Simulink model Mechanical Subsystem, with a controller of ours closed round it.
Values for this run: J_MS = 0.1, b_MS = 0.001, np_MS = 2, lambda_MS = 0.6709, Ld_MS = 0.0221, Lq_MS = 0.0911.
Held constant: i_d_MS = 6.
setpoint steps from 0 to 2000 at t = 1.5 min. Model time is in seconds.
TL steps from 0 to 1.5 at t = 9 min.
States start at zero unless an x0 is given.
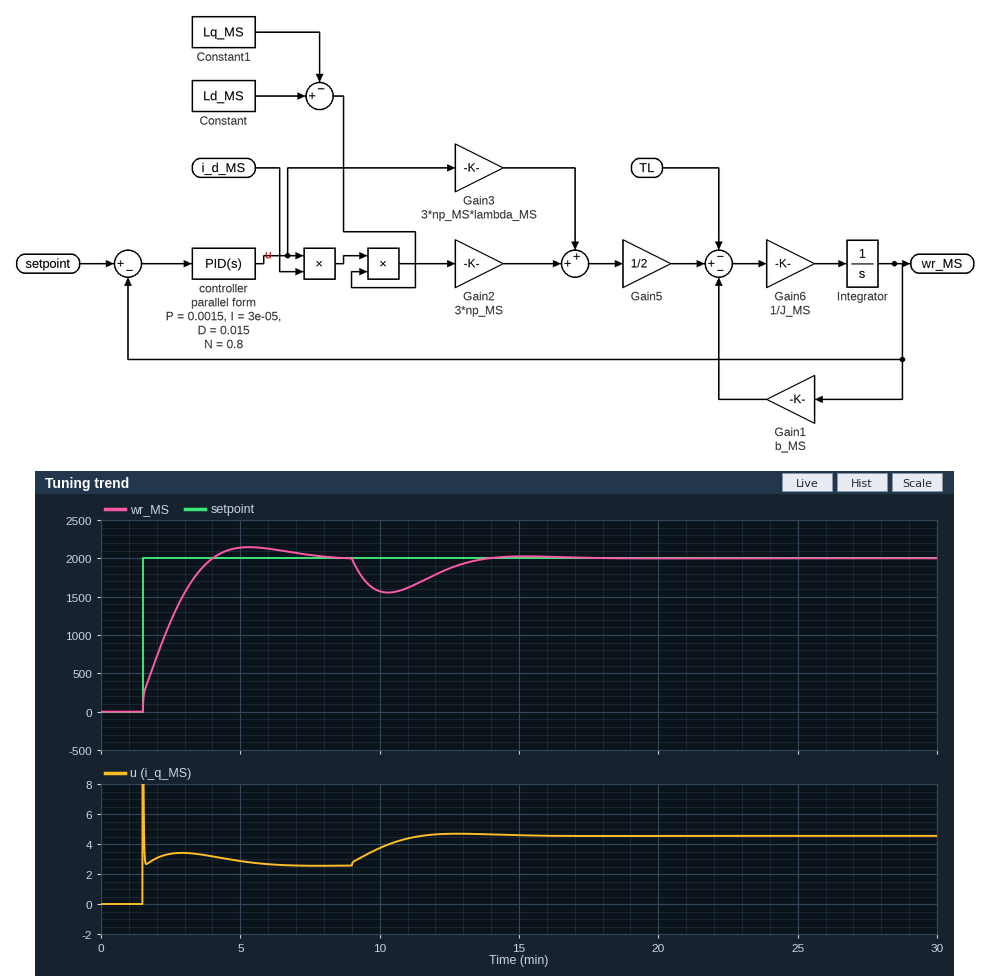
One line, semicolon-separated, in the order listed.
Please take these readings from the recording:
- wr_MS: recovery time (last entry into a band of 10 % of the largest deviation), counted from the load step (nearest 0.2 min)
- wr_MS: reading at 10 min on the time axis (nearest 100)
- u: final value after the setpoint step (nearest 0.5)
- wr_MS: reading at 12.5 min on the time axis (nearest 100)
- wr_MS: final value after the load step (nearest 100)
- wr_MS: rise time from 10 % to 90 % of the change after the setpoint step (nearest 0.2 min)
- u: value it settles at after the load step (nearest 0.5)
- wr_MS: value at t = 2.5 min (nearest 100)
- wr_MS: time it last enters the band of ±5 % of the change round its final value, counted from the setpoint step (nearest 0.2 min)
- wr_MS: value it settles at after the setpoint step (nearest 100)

4.2 min; 1600; 2.5; 1900; 2000; 2.0 min; 4.5; 1200; 5.0 min; 2000
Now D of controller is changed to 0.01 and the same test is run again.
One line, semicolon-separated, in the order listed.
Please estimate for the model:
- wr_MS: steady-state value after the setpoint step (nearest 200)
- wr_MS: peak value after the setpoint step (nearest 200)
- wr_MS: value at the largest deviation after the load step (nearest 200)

2000; 2200; 1600
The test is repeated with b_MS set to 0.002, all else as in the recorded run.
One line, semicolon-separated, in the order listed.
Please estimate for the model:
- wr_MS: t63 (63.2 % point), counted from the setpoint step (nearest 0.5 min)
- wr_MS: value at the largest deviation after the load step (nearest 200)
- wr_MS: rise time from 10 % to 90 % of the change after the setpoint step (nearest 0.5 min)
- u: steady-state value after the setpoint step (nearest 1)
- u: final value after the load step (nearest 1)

1.5 min; 1600; 3.5 min; 5; 7
